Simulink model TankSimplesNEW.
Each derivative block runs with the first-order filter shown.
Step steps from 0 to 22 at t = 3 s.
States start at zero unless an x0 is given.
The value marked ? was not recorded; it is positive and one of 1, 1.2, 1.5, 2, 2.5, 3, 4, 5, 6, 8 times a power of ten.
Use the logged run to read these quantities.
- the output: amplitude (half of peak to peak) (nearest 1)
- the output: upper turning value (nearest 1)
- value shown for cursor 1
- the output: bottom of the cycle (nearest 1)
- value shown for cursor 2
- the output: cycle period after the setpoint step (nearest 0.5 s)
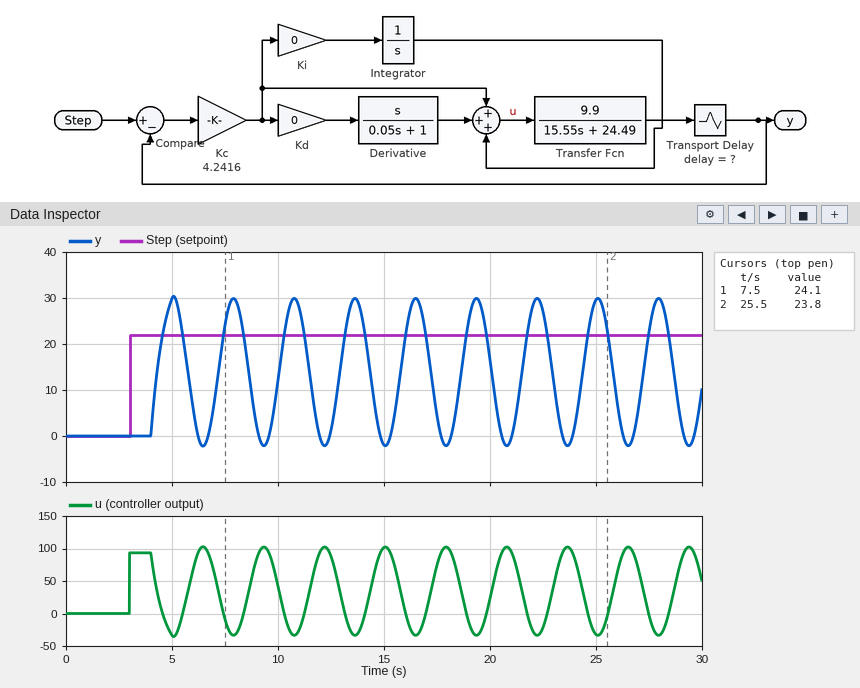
16
30
24.1
-2
23.8
3.0 s
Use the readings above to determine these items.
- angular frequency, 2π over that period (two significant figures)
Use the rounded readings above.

2.1 rad/s
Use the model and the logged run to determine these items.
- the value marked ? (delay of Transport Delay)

1
